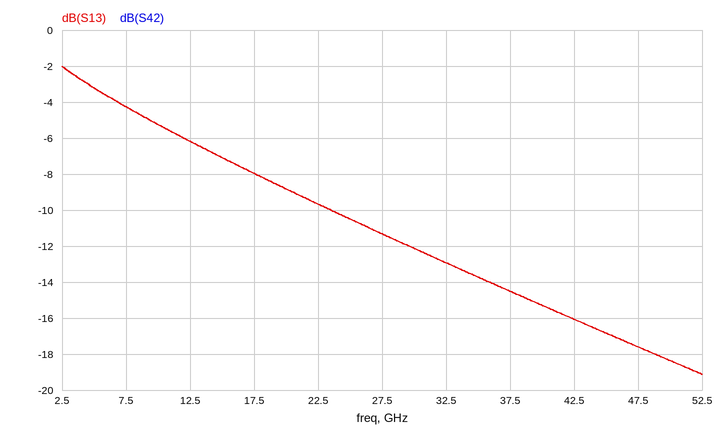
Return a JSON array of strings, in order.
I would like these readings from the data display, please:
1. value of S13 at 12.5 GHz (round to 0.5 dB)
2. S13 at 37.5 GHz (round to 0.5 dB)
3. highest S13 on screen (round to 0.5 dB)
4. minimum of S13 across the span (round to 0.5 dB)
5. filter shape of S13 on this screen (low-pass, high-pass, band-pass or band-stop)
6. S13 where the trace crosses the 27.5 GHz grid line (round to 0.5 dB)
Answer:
["-6.0 dB", "-14.5 dB", "-2.0 dB", "-19.0 dB", "low-pass", "-11.5 dB"]
